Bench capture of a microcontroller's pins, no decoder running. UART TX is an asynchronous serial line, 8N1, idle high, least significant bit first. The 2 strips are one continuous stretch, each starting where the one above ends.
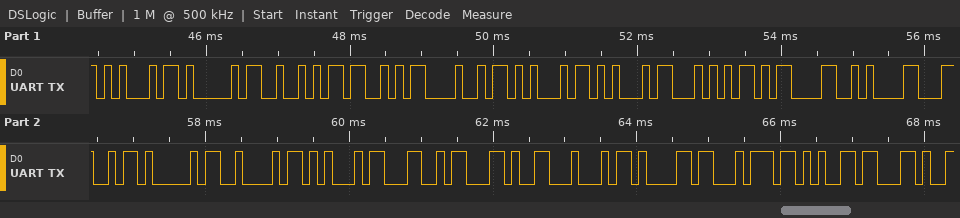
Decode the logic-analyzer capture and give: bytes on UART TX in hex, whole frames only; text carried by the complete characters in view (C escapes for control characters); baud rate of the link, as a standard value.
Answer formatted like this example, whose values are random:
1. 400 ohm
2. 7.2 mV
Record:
1. 0x45 0x41 0x52 0x53 0x48 0x45 0x45 0x54 0x0D 0x0A 0x4C 0x41 0x42 0x45 0x4C 0x2C 0x44 0x61 0x74 0x65 0x2C
2. "EARSHEET\r\nLABEL,Date,"
3. 9600 baud
